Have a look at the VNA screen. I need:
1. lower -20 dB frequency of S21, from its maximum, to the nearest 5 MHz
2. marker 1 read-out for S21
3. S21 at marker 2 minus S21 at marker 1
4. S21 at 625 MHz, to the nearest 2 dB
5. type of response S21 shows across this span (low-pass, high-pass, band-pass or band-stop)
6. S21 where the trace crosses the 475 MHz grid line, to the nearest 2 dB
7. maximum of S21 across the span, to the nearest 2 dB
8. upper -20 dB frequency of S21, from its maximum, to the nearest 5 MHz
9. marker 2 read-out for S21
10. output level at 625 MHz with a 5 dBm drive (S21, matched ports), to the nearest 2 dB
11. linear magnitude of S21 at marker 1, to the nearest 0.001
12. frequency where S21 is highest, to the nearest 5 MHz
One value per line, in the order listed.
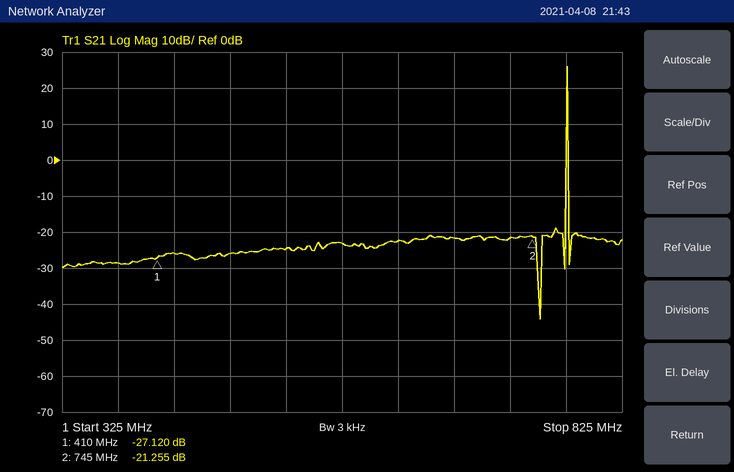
775 MHz
-27.120 dB
5.865 dB
-22 dB
band-pass
-26 dB
26 dB
775 MHz
-21.255 dB
-18 dBm
0.044
775 MHz
